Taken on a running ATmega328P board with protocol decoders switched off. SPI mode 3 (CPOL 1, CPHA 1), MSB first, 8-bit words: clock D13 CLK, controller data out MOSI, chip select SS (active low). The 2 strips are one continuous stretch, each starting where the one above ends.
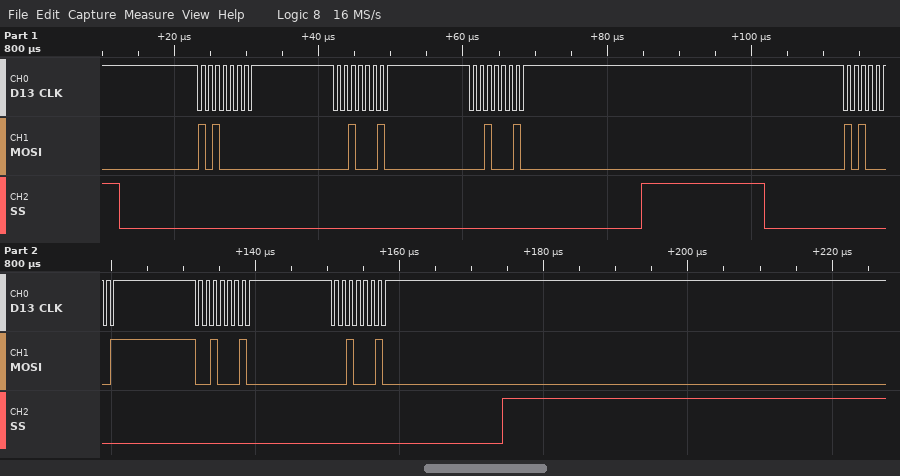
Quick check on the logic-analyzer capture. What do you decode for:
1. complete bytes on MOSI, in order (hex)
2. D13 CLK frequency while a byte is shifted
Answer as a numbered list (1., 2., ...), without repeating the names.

1. 0xA0 0x22 0x22 0xA1 0x22 0x22
2. 1 MHz
